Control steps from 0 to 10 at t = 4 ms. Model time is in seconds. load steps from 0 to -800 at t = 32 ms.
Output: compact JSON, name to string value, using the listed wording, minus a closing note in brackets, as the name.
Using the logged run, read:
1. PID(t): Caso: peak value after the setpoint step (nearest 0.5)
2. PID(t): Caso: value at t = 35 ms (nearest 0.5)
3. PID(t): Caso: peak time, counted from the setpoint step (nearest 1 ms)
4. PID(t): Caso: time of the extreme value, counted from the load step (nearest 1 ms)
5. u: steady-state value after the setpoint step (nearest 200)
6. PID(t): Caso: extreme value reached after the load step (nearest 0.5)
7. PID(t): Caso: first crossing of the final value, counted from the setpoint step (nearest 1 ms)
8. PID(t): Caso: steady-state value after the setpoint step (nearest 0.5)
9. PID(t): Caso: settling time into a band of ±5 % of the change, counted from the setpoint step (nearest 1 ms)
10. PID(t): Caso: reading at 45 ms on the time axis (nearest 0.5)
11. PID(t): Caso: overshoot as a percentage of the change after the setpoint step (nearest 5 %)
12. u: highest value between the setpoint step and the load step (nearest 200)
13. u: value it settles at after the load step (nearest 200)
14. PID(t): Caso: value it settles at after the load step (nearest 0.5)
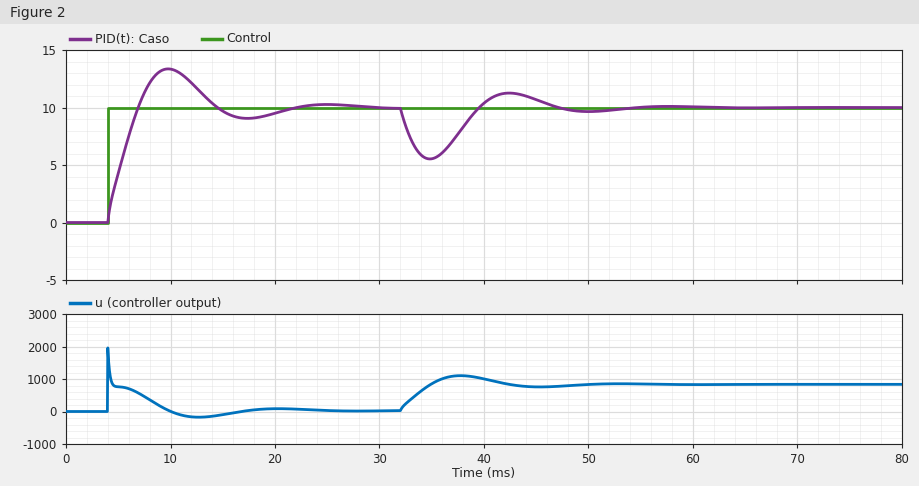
{"PID(t): Caso: peak value after the setpoint step": "13.5", "PID(t): Caso: value at t = 35 ms": "5.5", "PID(t): Caso: peak time, counted from the setpoint step": "6 ms", "PID(t): Caso: time of the extreme value, counted from the load step": "3 ms", "u: steady-state value after the setpoint step": "0", "PID(t): Caso: extreme value reached after the load step": "5.5", "PID(t): Caso: first crossing of the final value, counted from the setpoint step": "3 ms", "PID(t): Caso: steady-state value after the setpoint step": "10.0", "PID(t): Caso: settling time into a band of ±5 % of the change, counted from the setpoint step": "16 ms", "PID(t): Caso: reading at 45 ms on the time axis": "10.5", "PID(t): Caso: overshoot as a percentage of the change after the setpoint step": "35 %", "u: highest value between the setpoint step and the load step": "2000", "u: value it settles at after the load step": "800", "PID(t): Caso: value it settles at after the load step": "10.0"}
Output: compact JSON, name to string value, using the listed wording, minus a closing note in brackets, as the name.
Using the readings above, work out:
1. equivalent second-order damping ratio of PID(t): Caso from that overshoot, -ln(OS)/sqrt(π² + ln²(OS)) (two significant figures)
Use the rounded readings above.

{"equivalent second-order damping ratio of PID(t): Caso from that overshoot, -ln(OS)/sqrt(π² + ln²(OS))": "0.32"}
